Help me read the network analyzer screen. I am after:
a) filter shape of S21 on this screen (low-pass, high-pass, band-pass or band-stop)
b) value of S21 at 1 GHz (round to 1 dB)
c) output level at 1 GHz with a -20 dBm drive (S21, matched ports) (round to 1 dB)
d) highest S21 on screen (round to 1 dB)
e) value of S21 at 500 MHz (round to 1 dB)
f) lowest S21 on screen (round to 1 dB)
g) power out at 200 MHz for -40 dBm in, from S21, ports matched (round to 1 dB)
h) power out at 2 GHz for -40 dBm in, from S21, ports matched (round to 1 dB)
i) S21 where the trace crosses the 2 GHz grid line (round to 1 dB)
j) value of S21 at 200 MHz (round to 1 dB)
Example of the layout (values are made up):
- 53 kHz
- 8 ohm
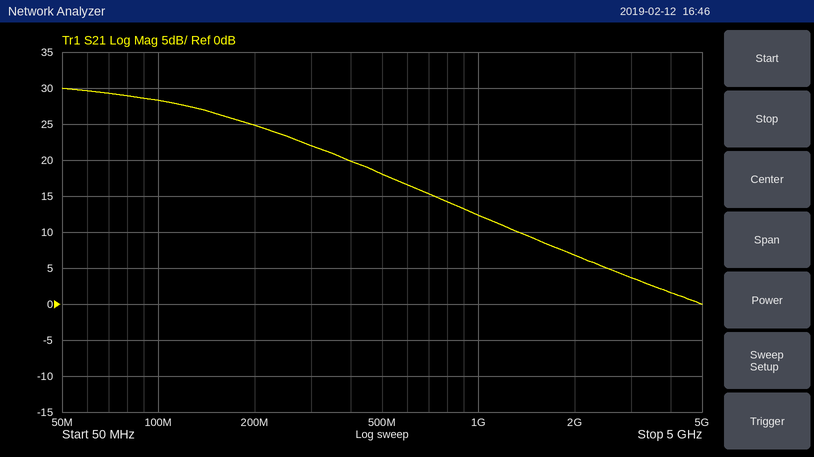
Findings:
- low-pass
- 12 dB
- -8 dBm
- 30 dB
- 18 dB
- 0 dB
- -15 dBm
- -33 dBm
- 7 dB
- 25 dB
